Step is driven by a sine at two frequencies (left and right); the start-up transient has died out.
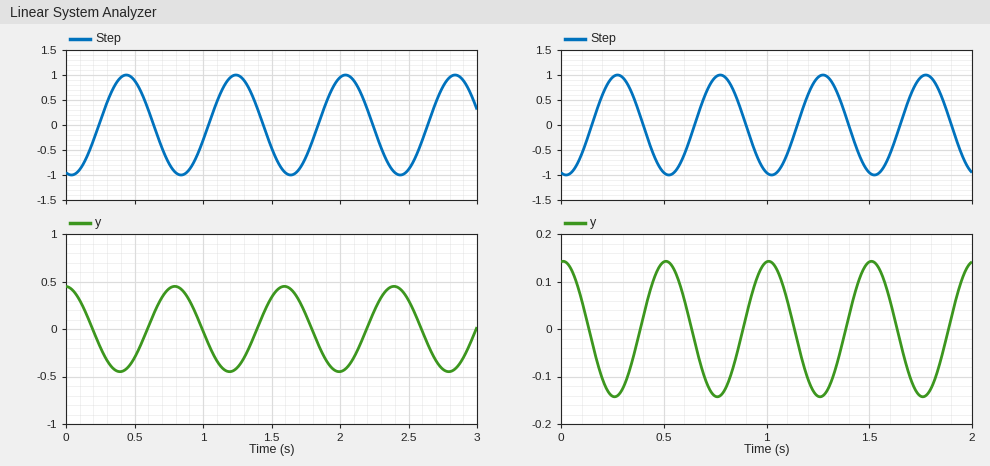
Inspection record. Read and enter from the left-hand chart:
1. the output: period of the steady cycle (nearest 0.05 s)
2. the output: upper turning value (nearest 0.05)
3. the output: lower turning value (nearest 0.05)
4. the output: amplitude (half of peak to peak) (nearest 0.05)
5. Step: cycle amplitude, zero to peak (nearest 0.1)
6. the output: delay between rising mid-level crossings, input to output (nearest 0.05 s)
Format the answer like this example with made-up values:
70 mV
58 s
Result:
0.80 s
0.45
-0.45
0.45
1.0
0.35 s
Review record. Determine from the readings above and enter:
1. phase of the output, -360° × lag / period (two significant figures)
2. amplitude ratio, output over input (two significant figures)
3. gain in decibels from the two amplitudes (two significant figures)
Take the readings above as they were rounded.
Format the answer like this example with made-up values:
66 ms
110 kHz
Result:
-160°
0.45
-6.9 dB
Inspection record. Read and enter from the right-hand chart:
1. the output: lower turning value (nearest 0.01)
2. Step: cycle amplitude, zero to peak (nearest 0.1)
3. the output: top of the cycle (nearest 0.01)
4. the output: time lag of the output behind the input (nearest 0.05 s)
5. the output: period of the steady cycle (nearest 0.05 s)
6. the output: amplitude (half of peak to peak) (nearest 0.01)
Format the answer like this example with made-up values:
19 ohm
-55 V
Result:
-0.14
1.0
0.14
0.25 s
0.50 s
0.14
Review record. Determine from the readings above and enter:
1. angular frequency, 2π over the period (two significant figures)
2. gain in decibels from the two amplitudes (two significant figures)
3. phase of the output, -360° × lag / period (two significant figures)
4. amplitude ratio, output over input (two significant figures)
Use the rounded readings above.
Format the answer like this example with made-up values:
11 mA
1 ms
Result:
13 rad/s
-17 dB
-180°
0.14
